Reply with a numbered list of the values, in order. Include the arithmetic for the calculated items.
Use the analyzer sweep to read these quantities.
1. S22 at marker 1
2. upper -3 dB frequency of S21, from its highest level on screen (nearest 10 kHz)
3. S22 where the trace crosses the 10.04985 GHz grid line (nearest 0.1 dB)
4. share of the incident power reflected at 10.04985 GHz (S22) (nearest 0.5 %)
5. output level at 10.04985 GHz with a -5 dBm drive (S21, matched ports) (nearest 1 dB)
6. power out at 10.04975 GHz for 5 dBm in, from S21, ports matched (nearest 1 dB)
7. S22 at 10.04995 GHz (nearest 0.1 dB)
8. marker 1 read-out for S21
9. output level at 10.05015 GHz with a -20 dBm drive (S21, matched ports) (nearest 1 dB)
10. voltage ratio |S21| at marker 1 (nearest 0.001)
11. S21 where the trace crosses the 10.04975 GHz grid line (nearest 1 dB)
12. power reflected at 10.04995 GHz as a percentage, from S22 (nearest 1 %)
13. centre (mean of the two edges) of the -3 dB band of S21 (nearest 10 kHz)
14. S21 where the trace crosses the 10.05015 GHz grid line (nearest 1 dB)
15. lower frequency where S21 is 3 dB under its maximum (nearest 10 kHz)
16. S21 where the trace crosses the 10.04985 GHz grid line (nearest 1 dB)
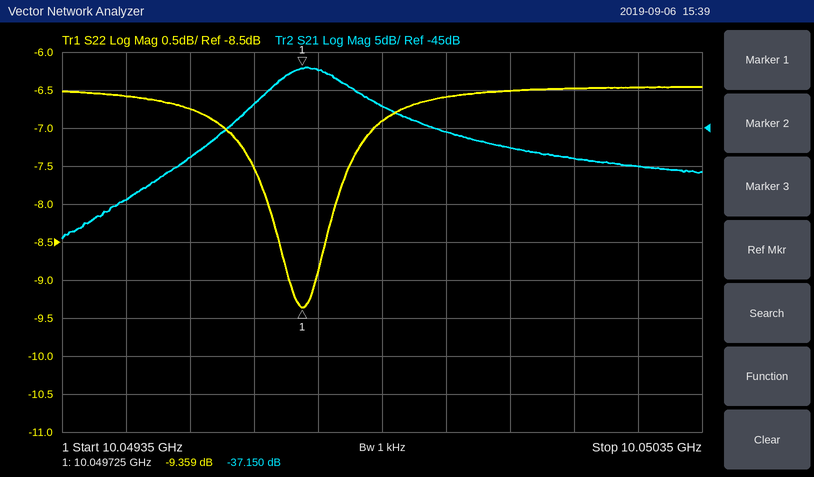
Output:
1. -9.359 dB
2. 10.04981 GHz
3. -6.9 dB
4. 10^(-6.9/10) ≈ 20.4 %, so 20.5 % to the nearest 0.5 %
5. -5 dBm + (-42 dB) = -47 dBm
6. 5 dBm + (-37 dB) = -32 dBm
7. -6.6 dB
8. -37.150 dB
9. -20 dBm + (-49 dB) = -69 dBm
10. 10^(-37.15/20) ≈ 0.014
11. -37 dB
12. 10^(-6.6/10) ≈ 22 %
13. 10.04974 GHz
14. -49 dB
15. 10.04967 GHz
16. -42 dB
